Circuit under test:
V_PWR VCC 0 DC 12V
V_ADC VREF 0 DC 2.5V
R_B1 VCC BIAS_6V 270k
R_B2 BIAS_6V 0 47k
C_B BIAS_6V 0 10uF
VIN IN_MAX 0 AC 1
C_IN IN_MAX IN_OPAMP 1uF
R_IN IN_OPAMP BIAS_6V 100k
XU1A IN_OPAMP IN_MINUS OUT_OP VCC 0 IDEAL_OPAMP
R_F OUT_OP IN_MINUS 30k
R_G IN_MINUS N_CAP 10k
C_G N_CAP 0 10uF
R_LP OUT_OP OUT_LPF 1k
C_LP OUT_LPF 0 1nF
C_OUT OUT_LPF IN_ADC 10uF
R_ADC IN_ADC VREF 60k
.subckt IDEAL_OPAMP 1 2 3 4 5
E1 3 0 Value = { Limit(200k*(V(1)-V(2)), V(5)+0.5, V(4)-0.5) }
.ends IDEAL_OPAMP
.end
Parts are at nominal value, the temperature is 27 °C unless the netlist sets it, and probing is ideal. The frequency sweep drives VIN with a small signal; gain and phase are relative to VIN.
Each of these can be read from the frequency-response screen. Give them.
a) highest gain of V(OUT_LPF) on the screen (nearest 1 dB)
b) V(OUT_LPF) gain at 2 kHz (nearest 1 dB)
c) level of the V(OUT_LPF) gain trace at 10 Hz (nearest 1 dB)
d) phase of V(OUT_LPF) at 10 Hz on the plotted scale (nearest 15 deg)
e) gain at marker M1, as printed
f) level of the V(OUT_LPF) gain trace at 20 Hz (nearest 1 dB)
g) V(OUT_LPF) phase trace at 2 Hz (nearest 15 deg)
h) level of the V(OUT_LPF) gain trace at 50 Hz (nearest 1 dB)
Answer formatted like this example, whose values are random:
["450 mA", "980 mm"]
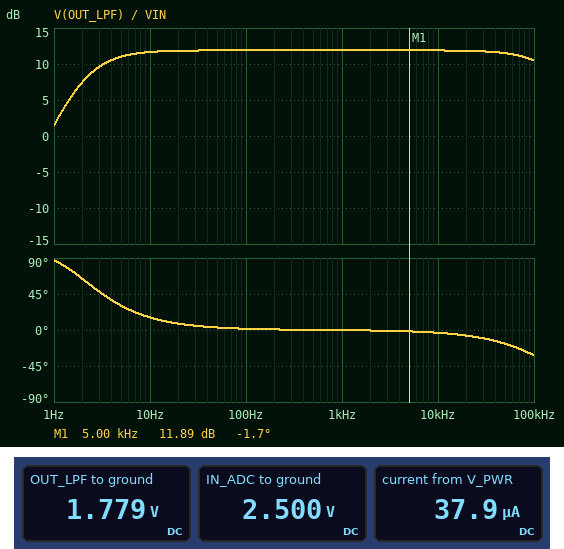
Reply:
["12 dB", "12 dB", "12 dB", "15 deg", "11.89 dB", "12 dB", "60 deg", "12 dB"]
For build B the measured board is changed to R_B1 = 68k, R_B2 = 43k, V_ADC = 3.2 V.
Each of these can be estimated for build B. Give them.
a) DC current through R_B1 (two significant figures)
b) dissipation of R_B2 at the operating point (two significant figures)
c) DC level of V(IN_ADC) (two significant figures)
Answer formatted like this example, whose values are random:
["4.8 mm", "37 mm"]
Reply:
["110 µA", "500 µW", "3.2 V"]
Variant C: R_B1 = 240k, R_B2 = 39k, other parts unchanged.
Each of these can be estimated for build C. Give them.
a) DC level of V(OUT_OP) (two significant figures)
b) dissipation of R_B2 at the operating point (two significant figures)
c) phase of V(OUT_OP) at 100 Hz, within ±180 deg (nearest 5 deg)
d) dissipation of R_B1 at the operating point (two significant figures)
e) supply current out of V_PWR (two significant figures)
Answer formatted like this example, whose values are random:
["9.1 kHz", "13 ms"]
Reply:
["1.7 V", "72 µW", "0 deg", "440 µW", "43 µA"]
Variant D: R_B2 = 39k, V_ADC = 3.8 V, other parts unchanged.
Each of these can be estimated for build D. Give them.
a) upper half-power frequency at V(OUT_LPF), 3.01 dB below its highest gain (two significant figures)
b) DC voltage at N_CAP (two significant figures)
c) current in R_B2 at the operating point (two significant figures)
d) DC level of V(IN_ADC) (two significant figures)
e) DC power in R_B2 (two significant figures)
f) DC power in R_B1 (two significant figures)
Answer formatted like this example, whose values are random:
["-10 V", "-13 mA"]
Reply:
["160 kHz", "1.5 V", "39 µA", "3.8 V", "59 µW", "410 µW"]
